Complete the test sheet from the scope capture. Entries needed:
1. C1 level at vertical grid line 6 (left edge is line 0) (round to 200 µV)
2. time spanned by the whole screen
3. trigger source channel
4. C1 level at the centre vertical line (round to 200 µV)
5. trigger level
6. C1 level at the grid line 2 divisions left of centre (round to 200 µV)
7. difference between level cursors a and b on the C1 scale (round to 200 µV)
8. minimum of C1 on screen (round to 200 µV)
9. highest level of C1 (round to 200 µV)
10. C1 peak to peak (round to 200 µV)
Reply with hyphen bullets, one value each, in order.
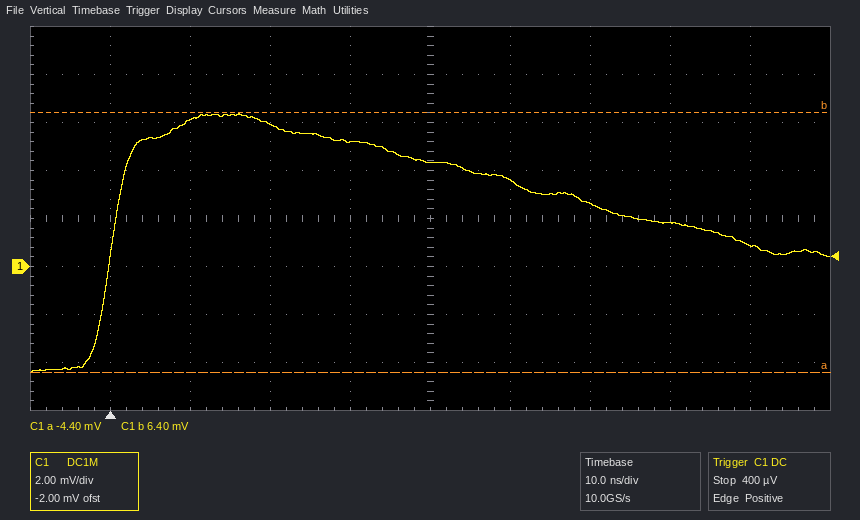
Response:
- 3.6 mV
- 100 ns
- C1
- 4.4 mV
- 400 µV
- 6.0 mV
- 10.8 mV
- -4.4 mV
- 6.4 mV
- 10.8 mV
